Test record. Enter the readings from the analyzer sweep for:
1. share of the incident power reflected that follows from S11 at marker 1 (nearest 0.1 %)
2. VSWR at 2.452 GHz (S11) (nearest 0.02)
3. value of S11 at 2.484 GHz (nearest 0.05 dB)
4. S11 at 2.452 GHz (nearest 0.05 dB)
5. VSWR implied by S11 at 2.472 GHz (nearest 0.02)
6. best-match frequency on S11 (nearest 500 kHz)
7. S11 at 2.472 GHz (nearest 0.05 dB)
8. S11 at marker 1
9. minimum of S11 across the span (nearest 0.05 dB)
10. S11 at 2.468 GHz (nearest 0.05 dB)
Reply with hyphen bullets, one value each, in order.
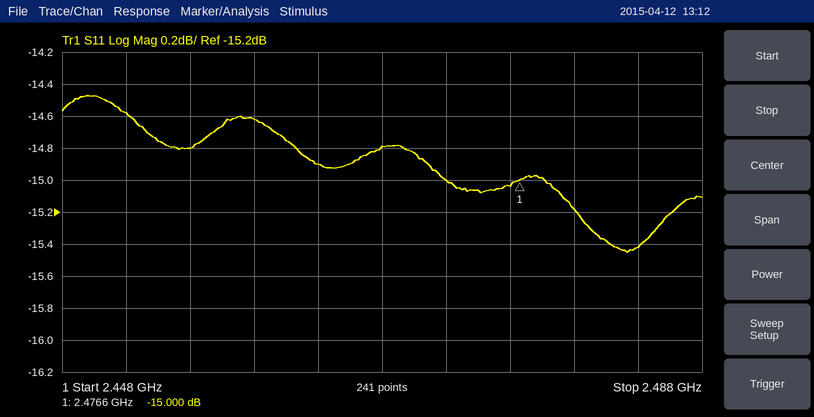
- 3.2 %
- 1.46
- -15.40 dB
- -14.60 dB
- 1.44
- 2.4835 GHz
- -15.00 dB
- -15.000 dB
- -15.45 dB
- -14.80 dB
